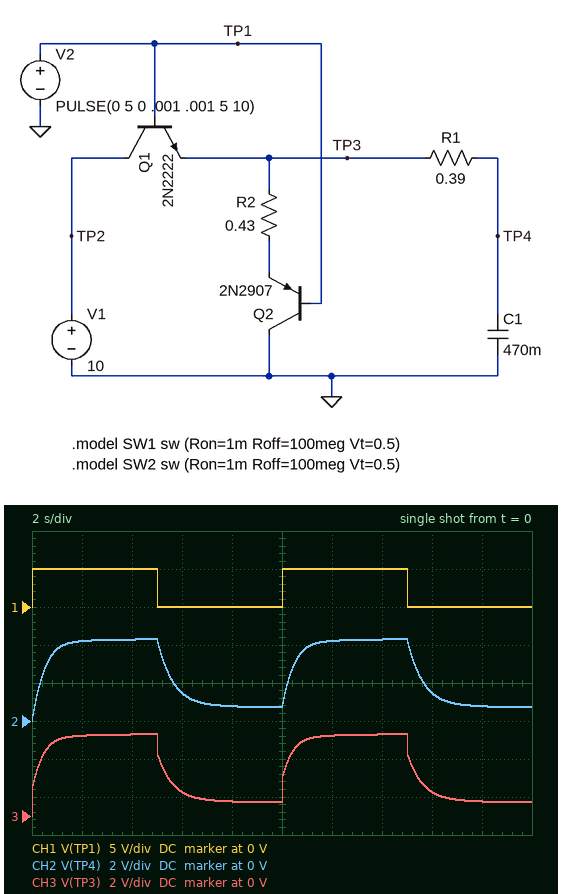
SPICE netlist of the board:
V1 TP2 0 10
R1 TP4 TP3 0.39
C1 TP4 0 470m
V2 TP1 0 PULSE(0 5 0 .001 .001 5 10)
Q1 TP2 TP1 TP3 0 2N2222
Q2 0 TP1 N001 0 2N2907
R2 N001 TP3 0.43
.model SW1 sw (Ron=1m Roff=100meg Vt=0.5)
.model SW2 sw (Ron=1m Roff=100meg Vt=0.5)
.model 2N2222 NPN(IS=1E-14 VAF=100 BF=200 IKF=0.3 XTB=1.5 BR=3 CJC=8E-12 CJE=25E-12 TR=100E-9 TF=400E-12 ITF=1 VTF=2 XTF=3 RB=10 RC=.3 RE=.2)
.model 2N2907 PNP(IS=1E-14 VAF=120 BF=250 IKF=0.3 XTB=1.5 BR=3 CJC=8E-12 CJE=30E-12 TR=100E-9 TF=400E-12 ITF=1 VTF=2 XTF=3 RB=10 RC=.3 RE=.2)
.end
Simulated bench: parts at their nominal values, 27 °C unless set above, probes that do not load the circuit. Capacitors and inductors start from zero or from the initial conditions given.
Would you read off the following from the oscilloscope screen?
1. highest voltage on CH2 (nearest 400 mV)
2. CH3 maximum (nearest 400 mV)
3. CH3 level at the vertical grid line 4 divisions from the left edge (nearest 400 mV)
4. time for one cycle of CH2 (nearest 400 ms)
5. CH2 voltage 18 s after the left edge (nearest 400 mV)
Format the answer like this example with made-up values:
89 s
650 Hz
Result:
4.4 V
4.4 V
800 mV
10.0 s
800 mV
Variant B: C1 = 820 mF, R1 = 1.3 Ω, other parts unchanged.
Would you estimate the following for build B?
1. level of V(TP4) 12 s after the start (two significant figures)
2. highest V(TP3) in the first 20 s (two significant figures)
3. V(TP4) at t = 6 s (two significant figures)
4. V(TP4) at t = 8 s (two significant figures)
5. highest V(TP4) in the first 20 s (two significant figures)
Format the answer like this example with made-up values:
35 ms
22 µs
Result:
3.4 V
4.2 V
2.7 V
1.4 V
4.1 V
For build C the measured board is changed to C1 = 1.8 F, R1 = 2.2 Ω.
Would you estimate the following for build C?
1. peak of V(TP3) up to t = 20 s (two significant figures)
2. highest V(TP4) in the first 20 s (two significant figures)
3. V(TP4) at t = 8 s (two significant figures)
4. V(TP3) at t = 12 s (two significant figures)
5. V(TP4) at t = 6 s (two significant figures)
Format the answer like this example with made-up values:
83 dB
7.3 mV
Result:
4.1 V
3.3 V
1.9 V
3.9 V
2.4 V
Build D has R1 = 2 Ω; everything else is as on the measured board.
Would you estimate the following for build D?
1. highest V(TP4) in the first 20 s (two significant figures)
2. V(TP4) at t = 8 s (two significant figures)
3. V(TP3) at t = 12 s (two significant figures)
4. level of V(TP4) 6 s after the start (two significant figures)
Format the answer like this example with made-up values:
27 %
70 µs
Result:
4.2 V
1.1 V
4.1 V
2.4 V
